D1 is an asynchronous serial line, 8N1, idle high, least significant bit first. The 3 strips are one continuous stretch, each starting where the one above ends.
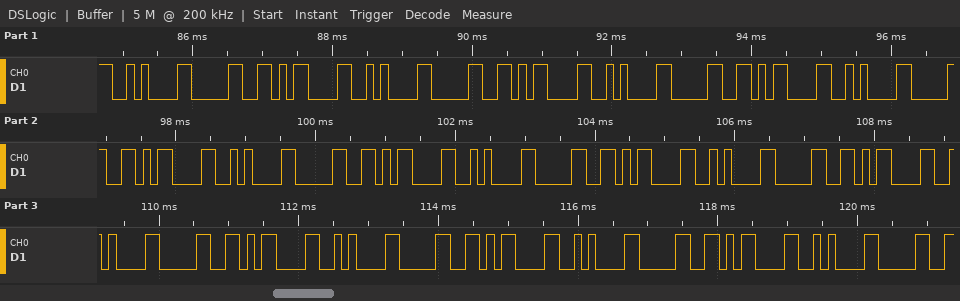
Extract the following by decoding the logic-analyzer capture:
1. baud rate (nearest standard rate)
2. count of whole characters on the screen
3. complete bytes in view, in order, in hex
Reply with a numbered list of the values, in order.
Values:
1. 9600 baud
2. 32
3. 0A 30 0D 0A 30 0D 0A 30 0D 0A 30 0D 0A 30 0D 0A 30 0D 0A 30 0D 0A 30 0D 0A 30 0D 0A 30 0D 0A 30
